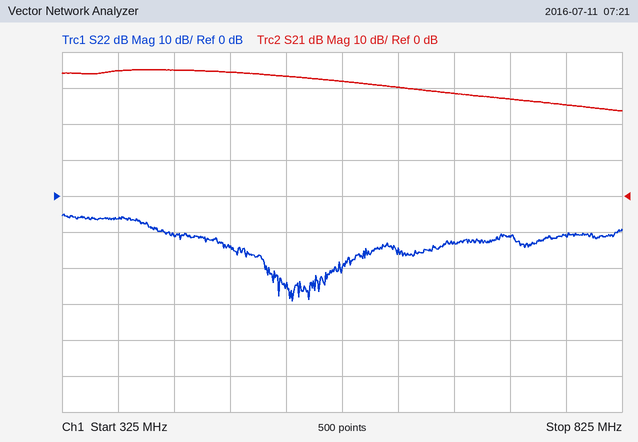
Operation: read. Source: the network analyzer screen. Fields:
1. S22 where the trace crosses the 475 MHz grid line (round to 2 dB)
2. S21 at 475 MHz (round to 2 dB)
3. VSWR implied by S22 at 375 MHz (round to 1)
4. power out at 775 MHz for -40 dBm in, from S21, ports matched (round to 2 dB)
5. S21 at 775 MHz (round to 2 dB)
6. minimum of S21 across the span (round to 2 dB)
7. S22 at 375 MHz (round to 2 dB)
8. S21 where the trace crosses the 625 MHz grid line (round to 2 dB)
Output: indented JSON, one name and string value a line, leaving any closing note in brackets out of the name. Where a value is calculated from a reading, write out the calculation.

{
  "S22 where the trace crosses the 475 MHz grid line": "-14 dB",
  "S21 at 475 MHz": "34 dB",
  "VSWR implied by S22 at 375 MHz": "|Γ| = 10^(-6/20) = 0.5012; VSWR = (1 + 0.5012)/(1 − 0.5012) ≈ 3",
  "power out at 775 MHz for -40 dBm in, from S21, ports matched": "-40 dBm + (26 dB) = -14 dBm",
  "S21 at 775 MHz": "26 dB",
  "minimum of S21 across the span": "24 dB",
  "S22 at 375 MHz": "-6 dB",
  "S21 where the trace crosses the 625 MHz grid line": "30 dB"
}
